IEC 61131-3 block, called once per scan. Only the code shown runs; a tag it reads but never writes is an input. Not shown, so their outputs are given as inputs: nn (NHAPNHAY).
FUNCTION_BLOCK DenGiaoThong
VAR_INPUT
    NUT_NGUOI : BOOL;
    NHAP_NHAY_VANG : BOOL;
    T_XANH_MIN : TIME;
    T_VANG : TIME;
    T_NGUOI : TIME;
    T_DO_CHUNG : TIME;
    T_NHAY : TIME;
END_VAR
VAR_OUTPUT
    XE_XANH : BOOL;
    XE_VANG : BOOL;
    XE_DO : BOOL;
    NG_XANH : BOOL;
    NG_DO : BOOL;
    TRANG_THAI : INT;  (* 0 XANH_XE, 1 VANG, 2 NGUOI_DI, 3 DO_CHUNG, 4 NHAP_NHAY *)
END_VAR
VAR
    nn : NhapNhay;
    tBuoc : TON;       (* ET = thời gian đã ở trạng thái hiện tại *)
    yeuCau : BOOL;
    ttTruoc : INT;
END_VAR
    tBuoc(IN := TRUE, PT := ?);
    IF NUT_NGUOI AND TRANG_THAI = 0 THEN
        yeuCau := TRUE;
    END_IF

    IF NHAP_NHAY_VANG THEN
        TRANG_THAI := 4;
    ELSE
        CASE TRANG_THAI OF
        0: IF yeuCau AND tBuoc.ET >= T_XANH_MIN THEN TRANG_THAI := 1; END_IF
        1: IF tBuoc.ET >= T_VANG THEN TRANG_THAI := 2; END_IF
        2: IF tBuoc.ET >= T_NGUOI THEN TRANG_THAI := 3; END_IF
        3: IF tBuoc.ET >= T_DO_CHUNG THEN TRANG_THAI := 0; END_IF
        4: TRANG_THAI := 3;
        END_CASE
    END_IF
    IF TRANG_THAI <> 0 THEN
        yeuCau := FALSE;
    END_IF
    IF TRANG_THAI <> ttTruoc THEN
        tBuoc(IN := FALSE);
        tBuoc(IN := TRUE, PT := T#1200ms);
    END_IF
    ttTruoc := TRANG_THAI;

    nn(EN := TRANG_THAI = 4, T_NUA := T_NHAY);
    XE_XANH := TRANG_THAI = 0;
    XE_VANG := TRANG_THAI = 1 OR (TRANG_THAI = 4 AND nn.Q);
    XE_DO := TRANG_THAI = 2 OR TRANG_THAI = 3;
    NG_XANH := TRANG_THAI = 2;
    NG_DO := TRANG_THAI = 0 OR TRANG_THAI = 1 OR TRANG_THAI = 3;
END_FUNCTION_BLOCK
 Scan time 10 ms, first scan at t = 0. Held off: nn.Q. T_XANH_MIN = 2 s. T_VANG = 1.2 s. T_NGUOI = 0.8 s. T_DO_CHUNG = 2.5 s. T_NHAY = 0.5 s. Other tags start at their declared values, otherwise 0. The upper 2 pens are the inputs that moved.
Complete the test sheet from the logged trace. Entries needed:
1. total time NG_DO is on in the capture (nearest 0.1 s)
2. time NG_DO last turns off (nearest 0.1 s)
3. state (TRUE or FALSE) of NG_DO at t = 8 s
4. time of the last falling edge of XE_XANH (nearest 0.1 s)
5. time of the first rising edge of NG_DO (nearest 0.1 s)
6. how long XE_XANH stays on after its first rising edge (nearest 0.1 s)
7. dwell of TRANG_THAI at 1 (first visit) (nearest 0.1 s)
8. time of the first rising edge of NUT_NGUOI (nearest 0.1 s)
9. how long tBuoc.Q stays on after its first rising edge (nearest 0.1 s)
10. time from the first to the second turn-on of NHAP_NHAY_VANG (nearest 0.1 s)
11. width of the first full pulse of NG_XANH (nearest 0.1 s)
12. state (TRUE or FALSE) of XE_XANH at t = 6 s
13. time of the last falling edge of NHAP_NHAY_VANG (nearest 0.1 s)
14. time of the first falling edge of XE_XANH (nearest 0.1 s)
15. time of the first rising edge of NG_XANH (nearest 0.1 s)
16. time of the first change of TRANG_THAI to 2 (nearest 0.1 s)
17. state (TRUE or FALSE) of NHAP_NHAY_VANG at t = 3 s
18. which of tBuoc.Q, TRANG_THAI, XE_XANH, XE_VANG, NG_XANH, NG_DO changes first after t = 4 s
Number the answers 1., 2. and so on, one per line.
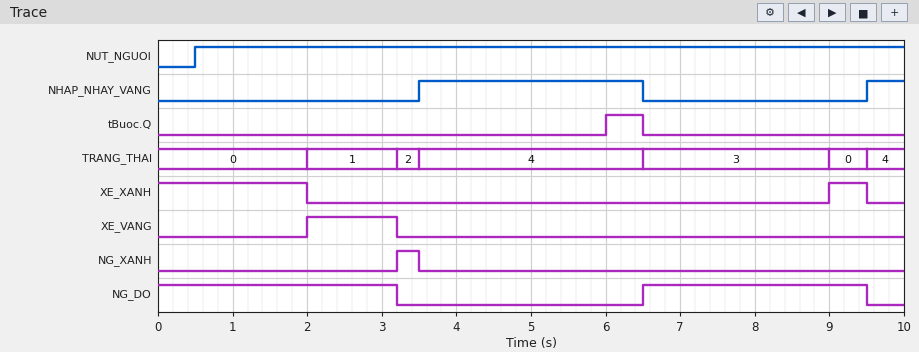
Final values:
1. 6.2 s
2. 9.5 s
3. TRUE
4. 9.5 s
5. 6.5 s
6. 0.5 s
7. 1.2 s
8. 0.5 s
9. 0.5 s
10. 6.0 s
11. 0.3 s
12. FALSE
13. 6.5 s
14. 2.0 s
15. 3.2 s
16. 3.2 s
17. FALSE
18. tBuoc.Q
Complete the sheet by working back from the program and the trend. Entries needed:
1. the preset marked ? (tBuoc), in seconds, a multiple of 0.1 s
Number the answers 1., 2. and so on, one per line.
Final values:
1. 2.5 s
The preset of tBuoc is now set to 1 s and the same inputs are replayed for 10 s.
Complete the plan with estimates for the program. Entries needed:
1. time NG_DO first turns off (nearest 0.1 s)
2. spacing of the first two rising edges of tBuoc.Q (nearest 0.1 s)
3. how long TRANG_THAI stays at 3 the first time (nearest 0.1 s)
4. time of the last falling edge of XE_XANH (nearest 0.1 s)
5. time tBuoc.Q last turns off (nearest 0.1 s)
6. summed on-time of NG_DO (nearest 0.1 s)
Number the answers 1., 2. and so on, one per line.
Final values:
1. 3.5 s
2. 3.5 s
3. 3.0 s
4. 3.5 s
5. 9.5 s
6. 6.5 s
